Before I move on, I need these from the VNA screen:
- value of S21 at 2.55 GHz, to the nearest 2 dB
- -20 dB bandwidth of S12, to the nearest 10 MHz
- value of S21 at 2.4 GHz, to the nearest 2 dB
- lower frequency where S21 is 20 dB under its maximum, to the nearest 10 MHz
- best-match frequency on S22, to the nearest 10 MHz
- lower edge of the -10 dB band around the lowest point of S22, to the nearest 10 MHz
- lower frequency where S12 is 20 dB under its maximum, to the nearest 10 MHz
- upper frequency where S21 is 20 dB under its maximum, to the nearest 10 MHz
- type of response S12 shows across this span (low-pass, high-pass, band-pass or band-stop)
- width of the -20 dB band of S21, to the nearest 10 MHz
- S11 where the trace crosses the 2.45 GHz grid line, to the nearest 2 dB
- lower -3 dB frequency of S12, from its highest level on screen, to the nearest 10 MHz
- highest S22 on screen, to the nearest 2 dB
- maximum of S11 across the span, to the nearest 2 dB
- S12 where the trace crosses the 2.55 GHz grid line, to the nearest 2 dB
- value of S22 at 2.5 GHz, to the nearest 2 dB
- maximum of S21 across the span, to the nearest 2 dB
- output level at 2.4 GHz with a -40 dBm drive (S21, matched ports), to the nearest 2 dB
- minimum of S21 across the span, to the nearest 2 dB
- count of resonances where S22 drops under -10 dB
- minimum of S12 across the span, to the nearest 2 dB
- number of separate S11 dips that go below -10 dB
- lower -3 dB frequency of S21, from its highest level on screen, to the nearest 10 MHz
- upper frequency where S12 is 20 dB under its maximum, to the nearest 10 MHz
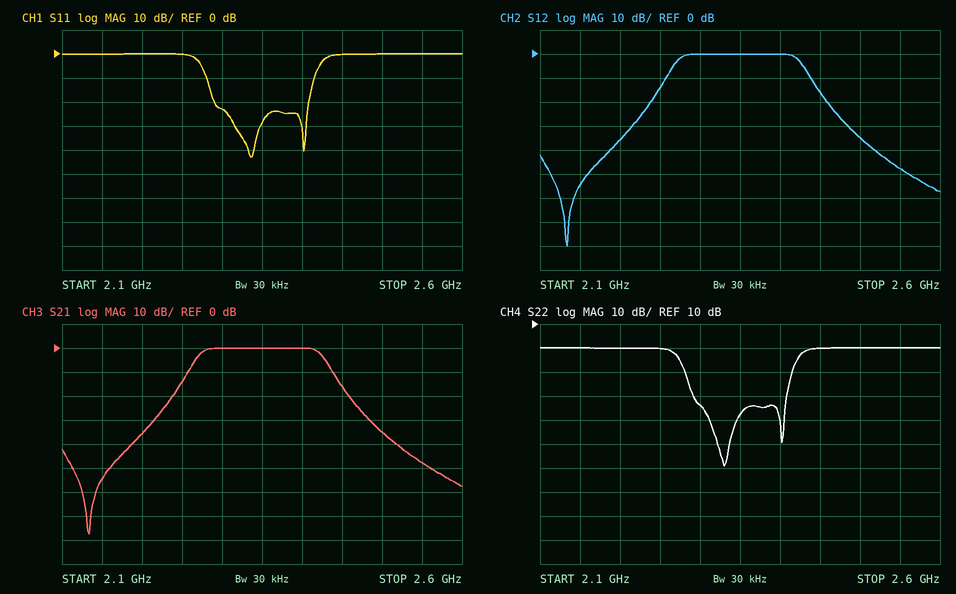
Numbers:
-48 dB
220 MHz
0 dB
2.24 GHz
2.33 GHz
2.28 GHz
2.24 GHz
2.46 GHz
band-pass
220 MHz
0 dB
2.27 GHz
0 dB
0 dB
-48 dB
0 dB
0 dB
-40 dBm
-78 dB
2
-80 dB
2
2.27 GHz
2.46 GHz
